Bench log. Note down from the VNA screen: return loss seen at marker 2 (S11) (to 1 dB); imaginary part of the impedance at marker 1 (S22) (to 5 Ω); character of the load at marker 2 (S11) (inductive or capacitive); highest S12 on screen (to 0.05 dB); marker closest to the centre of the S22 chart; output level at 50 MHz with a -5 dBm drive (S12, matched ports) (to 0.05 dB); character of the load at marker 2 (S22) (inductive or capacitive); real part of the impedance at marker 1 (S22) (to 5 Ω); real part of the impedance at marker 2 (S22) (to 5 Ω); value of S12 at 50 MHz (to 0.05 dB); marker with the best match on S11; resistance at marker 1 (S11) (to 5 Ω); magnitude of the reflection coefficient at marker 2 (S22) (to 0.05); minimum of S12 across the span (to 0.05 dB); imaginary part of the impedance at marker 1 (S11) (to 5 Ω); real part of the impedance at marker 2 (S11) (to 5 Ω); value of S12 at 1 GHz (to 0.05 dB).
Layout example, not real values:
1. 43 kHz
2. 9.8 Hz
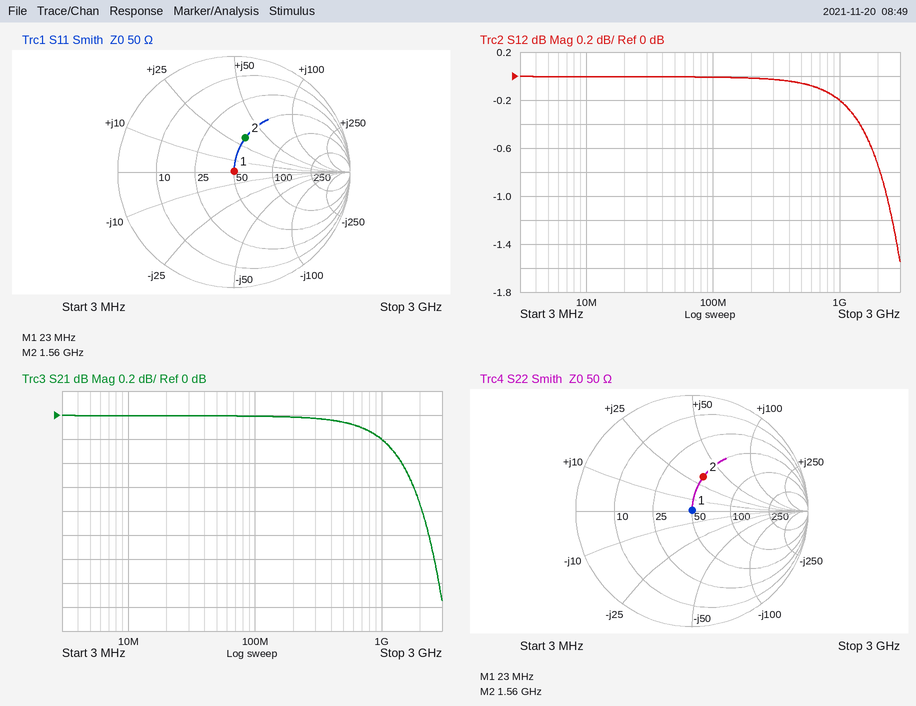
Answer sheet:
1. 10 dB
2. 0 Ω
3. inductive
4. 0.00 dB
5. marker 1
6. -5.00 dBm
7. inductive
8. 50 Ω
9. 50 Ω
10. 0.00 dB
11. marker 1
12. 50 Ω
13. 0.30
14. -1.55 dB
15. 0 Ω
16. 50 Ω
17. -0.20 dB
